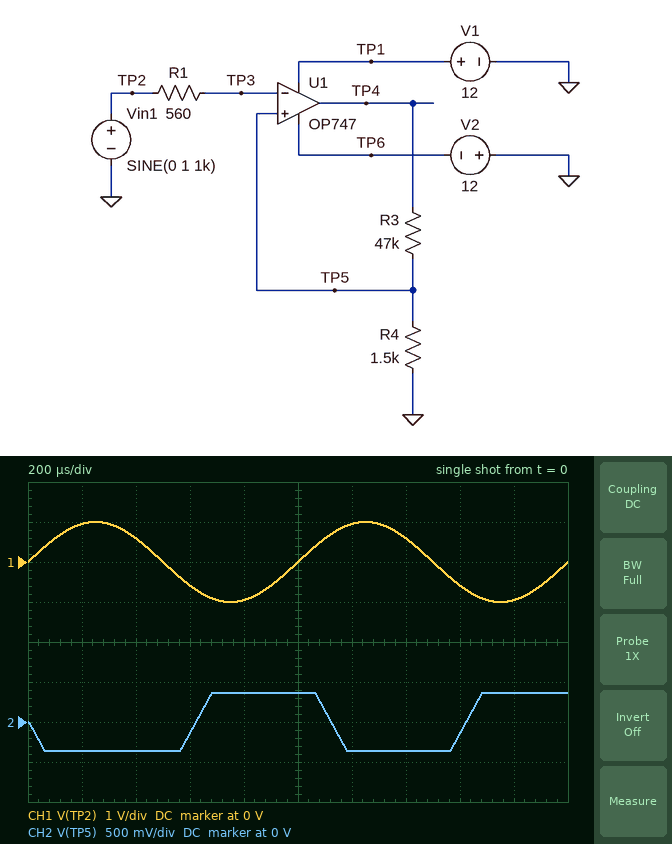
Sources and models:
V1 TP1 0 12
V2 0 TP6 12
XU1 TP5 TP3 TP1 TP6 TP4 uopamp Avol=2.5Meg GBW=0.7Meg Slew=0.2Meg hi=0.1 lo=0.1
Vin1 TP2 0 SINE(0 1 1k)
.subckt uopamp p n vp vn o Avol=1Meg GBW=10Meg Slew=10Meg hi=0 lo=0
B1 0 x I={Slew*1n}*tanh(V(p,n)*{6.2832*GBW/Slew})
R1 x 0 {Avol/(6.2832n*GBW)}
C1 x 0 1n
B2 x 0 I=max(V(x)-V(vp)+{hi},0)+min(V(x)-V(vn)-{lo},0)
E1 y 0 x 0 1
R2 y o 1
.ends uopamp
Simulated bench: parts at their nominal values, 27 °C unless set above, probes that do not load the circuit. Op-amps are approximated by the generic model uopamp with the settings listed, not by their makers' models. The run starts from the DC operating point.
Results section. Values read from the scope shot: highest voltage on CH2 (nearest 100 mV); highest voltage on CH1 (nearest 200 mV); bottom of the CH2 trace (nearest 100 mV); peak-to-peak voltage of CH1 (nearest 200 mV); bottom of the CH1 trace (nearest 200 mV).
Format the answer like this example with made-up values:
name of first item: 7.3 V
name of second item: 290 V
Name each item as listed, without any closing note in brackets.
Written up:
highest voltage on CH2: 400 mV
highest voltage on CH1: 1.0 V
bottom of the CH2 trace: -400 mV
peak-to-peak voltage of CH1: 2.0 V
bottom of the CH1 trace: -1.0 V
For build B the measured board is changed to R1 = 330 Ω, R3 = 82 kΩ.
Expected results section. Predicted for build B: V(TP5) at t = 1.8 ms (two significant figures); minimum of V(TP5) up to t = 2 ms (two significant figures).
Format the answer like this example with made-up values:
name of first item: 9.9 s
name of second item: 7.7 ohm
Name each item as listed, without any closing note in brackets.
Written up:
V(TP5) at t = 1.8 ms: 210 mV
minimum of V(TP5) up to t = 2 ms: -210 mV
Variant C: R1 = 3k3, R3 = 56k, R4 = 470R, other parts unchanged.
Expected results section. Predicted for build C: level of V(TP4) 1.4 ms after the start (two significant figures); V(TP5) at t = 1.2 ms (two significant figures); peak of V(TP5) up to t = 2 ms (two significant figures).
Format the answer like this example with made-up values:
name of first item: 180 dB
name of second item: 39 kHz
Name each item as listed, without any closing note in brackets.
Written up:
level of V(TP4) 1.4 ms after the start: -12 V
V(TP5) at t = 1.2 ms: -99 mV
peak of V(TP5) up to t = 2 ms: 99 mV
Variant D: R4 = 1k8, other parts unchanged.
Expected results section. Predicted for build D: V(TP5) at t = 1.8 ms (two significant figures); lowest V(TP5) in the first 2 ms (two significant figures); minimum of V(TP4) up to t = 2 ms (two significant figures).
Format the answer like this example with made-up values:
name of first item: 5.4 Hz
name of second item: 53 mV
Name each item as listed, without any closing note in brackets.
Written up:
V(TP5) at t = 1.8 ms: 440 mV
lowest V(TP5) in the first 2 ms: -440 mV
minimum of V(TP4) up to t = 2 ms: -12 V
